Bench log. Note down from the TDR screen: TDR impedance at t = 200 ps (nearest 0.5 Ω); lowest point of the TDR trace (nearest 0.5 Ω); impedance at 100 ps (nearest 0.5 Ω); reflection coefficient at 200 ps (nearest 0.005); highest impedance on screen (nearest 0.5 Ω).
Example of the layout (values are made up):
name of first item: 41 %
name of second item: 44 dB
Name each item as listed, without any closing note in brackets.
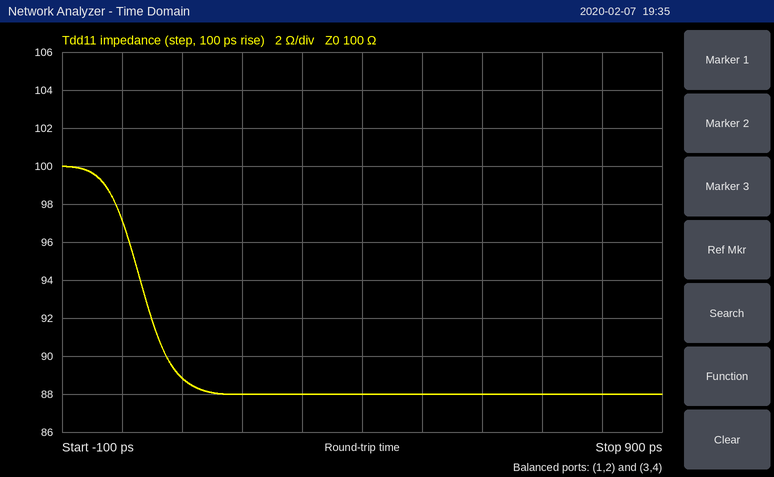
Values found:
TDR impedance at t = 200 ps: 88.0 Ω
lowest point of the TDR trace: 88.0 Ω
impedance at 100 ps: 89.0 Ω
reflection coefficient at 200 ps: -0.065
highest impedance on screen: 100.0 Ω
